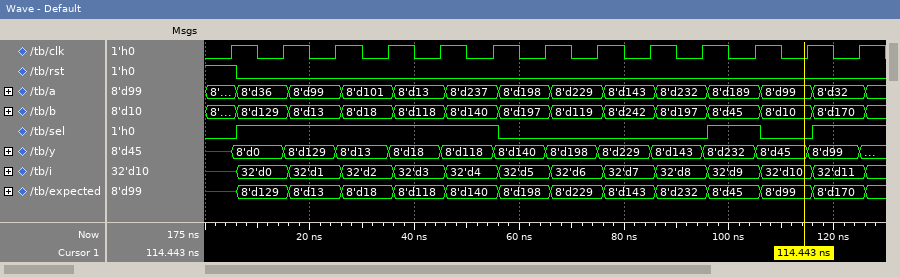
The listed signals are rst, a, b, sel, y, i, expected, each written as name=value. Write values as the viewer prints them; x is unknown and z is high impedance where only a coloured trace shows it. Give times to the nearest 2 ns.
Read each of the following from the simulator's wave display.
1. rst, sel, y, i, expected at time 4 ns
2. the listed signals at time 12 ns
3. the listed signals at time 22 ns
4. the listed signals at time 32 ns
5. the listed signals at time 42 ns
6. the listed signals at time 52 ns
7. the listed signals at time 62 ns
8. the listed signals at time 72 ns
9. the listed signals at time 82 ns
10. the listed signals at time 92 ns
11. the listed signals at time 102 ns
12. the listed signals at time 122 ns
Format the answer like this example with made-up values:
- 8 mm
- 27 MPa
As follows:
- rst=1, sel=0, y=x, i=x, expected=x
- rst=0, a=8'd36, b=8'd129, sel=1, y=8'd0, i=32'd0, expected=8'd129
- rst=0, a=8'd99, b=8'd13, sel=1, y=8'd129, i=32'd1, expected=8'd13
- rst=0, a=8'd101, b=8'd18, sel=1, y=8'd13, i=32'd2, expected=8'd18
- rst=0, a=8'd13, b=8'd118, sel=1, y=8'd18, i=32'd3, expected=8'd118
- rst=0, a=8'd237, b=8'd140, sel=1, y=8'd118, i=32'd4, expected=8'd140
- rst=0, a=8'd198, b=8'd197, sel=0, y=8'd140, i=32'd5, expected=8'd198
- rst=0, a=8'd229, b=8'd119, sel=0, y=8'd198, i=32'd6, expected=8'd229
- rst=0, a=8'd143, b=8'd242, sel=0, y=8'd229, i=32'd7, expected=8'd143
- rst=0, a=8'd232, b=8'd197, sel=0, y=8'd143, i=32'd8, expected=8'd232
- rst=0, a=8'd189, b=8'd45, sel=1, y=8'd232, i=32'd9, expected=8'd45
- rst=0, a=8'd32, b=8'd170, sel=1, y=8'd99, i=32'd11, expected=8'd170
